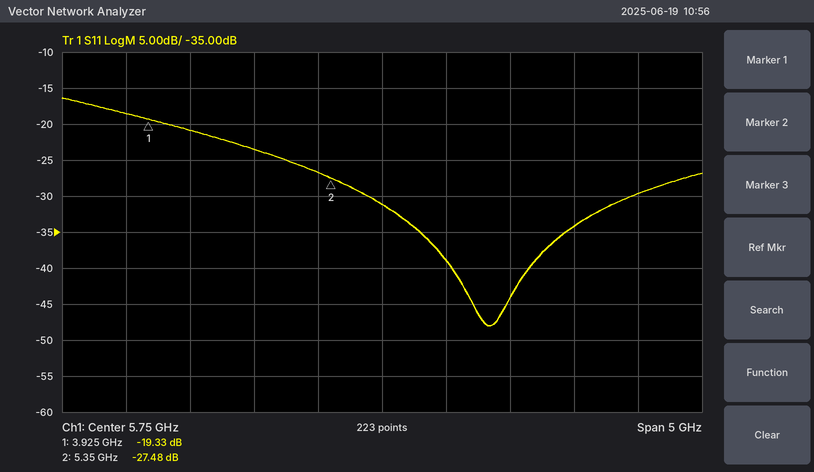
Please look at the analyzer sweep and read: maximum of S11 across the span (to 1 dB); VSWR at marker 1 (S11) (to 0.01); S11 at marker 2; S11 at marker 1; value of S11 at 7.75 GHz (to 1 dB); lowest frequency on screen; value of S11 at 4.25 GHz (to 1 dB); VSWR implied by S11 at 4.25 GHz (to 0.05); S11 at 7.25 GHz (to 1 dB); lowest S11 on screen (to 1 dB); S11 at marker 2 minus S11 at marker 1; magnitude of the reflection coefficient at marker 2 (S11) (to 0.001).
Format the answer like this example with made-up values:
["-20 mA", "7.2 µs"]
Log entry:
["-16 dB", "1.24", "-27.48 dB", "-19.33 dB", "-30 dB", "3.25 GHz", "-21 dB", "1.20", "-34 dB", "-48 dB", "-8.15 dB", "0.042"]
